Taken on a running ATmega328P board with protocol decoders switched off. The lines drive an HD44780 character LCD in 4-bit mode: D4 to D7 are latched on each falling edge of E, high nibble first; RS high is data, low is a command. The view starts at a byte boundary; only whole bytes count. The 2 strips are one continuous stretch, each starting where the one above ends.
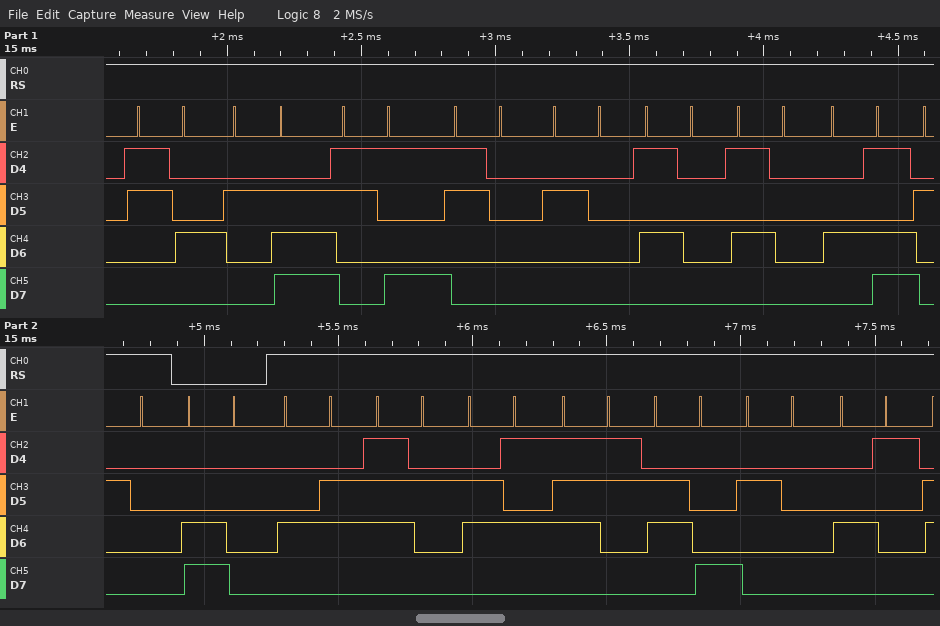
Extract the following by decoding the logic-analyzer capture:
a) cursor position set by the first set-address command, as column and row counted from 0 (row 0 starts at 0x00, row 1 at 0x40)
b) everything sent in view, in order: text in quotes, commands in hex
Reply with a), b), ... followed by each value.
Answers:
a) column 0, row 1
b) "4.90 PPM " 0xC0 "Fresh A"
